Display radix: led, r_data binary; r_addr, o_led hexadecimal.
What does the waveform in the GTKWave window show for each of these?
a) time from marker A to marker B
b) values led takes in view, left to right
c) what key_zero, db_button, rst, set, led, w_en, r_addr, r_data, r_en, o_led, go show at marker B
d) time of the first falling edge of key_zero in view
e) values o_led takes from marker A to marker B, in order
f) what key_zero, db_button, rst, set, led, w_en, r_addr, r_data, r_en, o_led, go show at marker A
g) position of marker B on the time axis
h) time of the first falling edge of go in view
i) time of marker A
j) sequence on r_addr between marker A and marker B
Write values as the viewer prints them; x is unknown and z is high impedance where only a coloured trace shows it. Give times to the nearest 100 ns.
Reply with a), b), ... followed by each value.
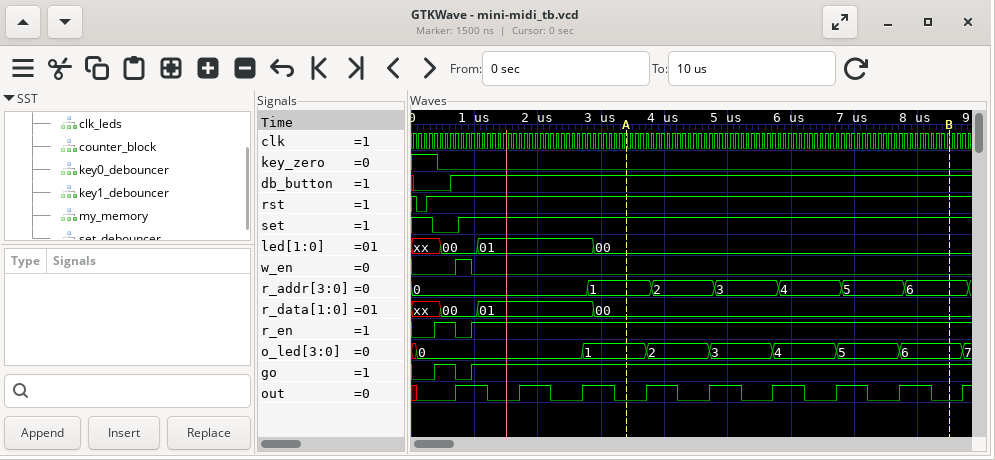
a) 5100 ns
b) xx, 00, 01, 00
c) key_zero=0, db_button=1, rst=1, set=1, led=00, w_en=0, r_addr=6, r_data=00, r_en=1, o_led=6, go=1
d) 400 ns
e) 1, 2, 3, 4, 5, 6
f) key_zero=0, db_button=1, rst=1, set=1, led=00, w_en=0, r_addr=1, r_data=00, r_en=1, o_led=1, go=1
g) 8500 ns
h) 700 ns
i) 3400 ns
j) 1, 2, 3, 4, 5, 6
